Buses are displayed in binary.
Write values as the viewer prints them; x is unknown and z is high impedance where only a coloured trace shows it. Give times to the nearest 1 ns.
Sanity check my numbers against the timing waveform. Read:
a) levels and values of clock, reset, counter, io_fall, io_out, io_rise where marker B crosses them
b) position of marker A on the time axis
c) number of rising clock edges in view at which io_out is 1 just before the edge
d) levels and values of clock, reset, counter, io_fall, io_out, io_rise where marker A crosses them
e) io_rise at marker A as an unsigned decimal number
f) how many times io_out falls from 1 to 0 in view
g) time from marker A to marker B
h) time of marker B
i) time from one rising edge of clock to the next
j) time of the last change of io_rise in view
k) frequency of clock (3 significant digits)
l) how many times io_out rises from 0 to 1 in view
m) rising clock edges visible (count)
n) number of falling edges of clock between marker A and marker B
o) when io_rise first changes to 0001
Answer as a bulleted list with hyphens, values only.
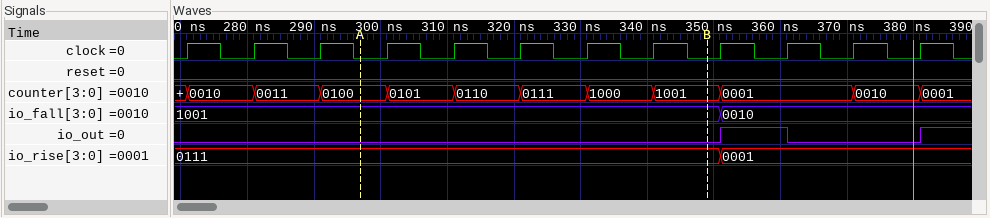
- clock=0, reset=0, counter=1001, io_fall=1001, io_out=0, io_rise=0111
- 297 ns
- 1
- clock=0, reset=0, counter=0100, io_fall=1001, io_out=0, io_rise=0111
- 7
- 1
- 52 ns
- 349 ns
- 10 ns
- 351 ns
- 100 MHz
- 2
- 12
- 5
- 351 ns
